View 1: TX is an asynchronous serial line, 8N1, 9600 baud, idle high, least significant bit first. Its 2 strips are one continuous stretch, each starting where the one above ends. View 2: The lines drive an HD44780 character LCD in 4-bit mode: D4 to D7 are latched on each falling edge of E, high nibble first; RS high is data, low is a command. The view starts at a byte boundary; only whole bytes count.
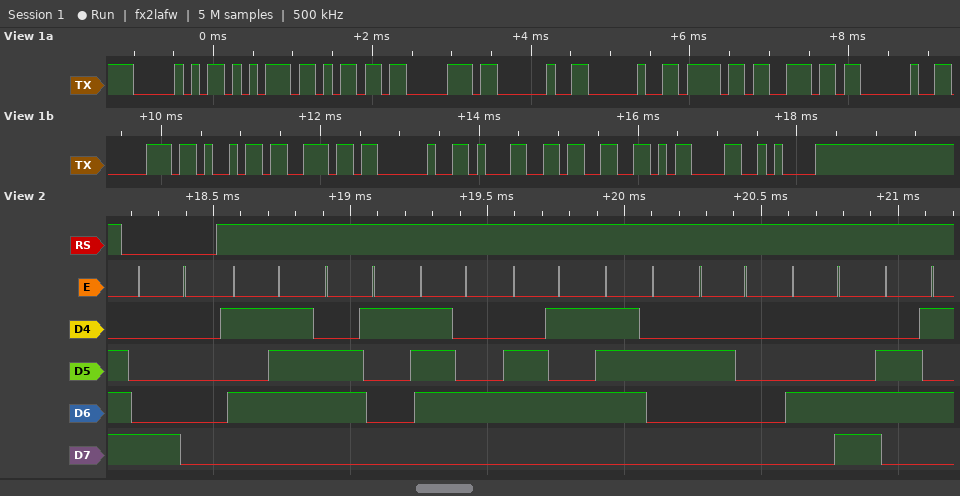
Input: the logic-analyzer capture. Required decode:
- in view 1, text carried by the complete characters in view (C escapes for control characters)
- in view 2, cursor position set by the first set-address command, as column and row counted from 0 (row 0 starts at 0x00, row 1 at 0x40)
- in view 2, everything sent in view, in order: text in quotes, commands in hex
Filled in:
"Pump  on pin 13\r\n"
column 0, row 0
0x80 "Water Le"
